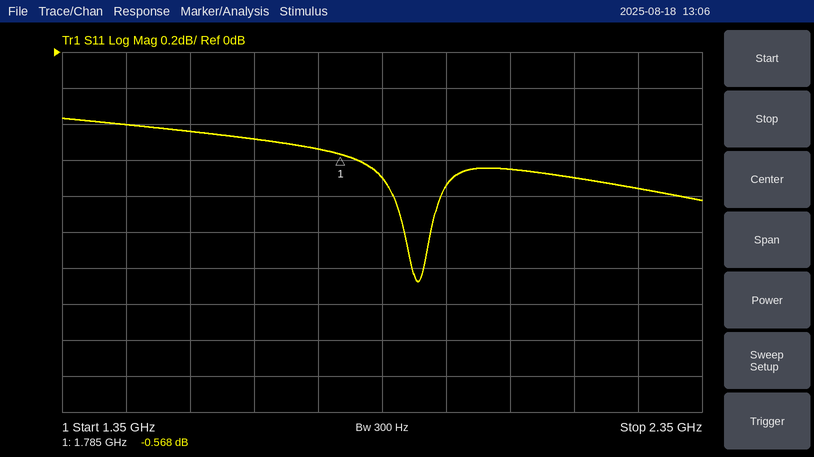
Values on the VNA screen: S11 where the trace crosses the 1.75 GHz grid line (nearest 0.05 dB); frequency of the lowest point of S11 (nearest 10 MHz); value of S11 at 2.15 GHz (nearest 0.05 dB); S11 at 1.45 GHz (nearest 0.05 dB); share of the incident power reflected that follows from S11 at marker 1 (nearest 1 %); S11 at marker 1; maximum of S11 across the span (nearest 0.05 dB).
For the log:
-0.55 dB
1.91 GHz
-0.70 dB
-0.40 dB
88 %
-0.568 dB
-0.35 dB
